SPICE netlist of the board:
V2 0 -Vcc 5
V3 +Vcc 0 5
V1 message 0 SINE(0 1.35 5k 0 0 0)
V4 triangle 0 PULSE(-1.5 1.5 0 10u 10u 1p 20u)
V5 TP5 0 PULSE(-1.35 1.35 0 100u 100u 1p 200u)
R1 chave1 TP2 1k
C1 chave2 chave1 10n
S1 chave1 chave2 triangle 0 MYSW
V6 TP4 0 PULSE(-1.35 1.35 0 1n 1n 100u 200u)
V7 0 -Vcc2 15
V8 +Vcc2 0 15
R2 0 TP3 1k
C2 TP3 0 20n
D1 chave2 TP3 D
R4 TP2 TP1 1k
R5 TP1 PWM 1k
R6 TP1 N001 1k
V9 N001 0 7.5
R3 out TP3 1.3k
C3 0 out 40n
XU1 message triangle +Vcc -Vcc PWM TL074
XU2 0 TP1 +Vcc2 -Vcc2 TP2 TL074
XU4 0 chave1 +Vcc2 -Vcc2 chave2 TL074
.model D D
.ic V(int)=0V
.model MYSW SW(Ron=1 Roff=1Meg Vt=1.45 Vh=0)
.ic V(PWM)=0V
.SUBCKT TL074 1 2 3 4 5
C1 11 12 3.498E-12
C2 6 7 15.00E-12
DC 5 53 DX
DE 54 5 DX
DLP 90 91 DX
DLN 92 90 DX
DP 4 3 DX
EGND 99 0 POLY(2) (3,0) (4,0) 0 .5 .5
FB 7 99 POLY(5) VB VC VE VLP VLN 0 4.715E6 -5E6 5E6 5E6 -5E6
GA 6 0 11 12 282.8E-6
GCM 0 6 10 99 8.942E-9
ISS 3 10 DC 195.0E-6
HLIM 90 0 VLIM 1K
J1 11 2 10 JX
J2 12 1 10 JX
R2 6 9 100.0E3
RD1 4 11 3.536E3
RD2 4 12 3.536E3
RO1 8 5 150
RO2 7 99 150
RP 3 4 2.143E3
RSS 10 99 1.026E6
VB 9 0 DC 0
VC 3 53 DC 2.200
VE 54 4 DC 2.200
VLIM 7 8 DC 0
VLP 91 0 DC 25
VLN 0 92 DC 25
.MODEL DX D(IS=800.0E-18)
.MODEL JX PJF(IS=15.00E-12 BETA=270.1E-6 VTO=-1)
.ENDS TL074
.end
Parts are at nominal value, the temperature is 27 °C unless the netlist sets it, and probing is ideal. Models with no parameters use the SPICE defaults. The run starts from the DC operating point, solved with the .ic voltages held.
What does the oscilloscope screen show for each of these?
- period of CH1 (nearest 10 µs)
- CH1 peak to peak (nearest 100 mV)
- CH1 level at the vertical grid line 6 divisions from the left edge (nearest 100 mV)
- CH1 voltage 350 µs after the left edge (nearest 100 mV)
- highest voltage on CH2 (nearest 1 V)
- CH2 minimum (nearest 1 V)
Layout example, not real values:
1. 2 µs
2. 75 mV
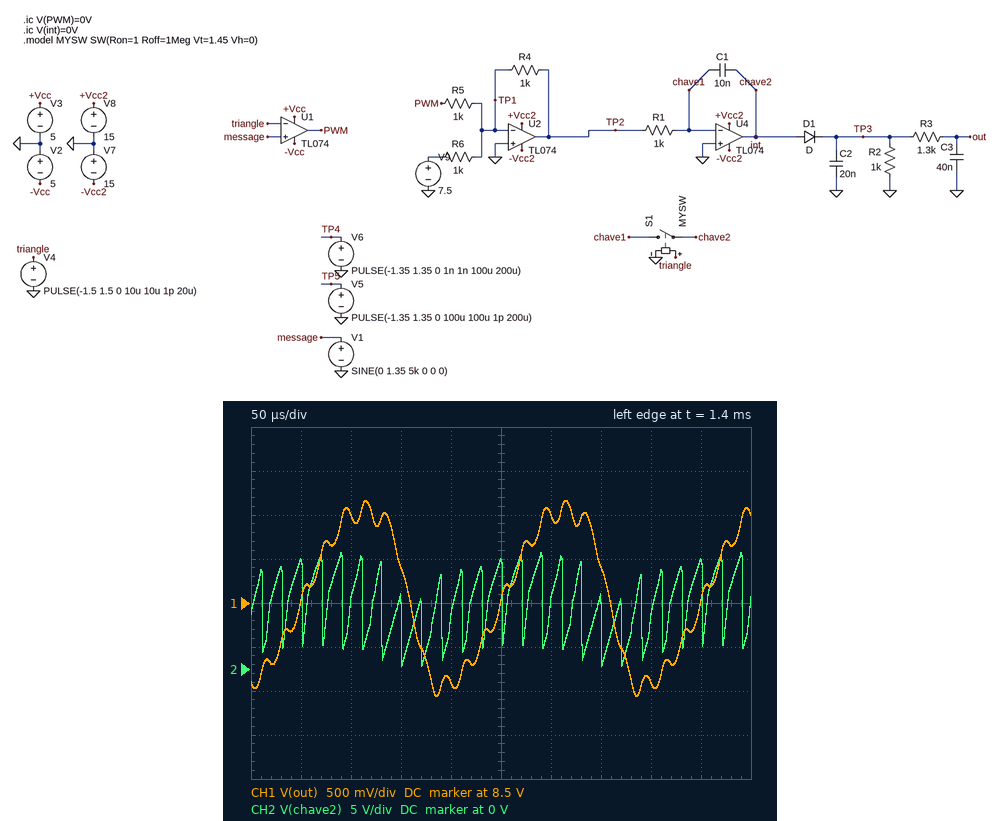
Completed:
1. 200 µs
2. 2.2 V
3. 9.5 V
4. 8.9 V
5. 13 V
6. 0 V
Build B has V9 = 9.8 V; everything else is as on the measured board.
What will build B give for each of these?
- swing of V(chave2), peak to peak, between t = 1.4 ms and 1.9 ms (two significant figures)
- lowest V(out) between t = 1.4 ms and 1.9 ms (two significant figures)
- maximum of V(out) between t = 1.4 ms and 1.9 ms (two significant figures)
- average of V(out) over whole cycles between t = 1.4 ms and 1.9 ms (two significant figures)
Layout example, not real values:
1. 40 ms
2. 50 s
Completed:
1. 11 V
2. 9.5 V
3. 10 V
4. 9.9 V
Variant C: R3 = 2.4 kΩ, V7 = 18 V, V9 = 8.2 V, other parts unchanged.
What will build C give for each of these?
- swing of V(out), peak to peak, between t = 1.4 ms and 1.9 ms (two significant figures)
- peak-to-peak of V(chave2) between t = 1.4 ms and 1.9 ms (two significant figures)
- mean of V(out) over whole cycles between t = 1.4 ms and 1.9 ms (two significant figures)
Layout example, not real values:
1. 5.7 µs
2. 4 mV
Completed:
1. 1.1 V
2. 13 V
3. 9.2 V
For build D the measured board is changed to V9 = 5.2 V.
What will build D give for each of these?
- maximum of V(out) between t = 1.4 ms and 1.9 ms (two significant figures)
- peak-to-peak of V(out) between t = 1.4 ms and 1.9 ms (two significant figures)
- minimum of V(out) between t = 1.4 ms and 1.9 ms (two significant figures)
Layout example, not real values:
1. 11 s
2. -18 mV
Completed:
1. 8.5 V
2. 3.6 V
3. 4.9 V
